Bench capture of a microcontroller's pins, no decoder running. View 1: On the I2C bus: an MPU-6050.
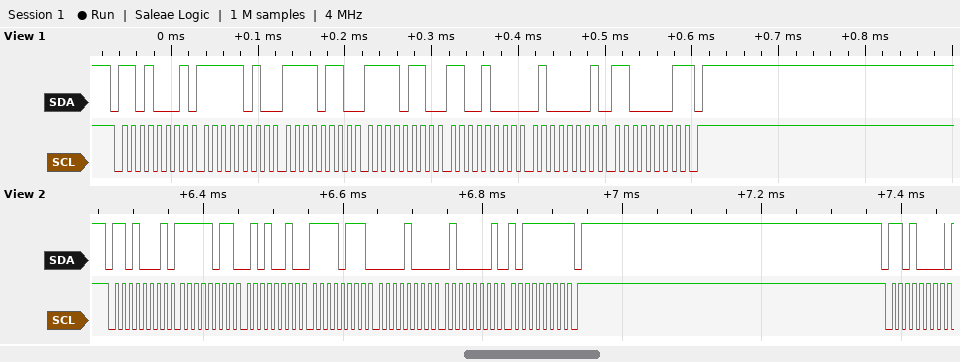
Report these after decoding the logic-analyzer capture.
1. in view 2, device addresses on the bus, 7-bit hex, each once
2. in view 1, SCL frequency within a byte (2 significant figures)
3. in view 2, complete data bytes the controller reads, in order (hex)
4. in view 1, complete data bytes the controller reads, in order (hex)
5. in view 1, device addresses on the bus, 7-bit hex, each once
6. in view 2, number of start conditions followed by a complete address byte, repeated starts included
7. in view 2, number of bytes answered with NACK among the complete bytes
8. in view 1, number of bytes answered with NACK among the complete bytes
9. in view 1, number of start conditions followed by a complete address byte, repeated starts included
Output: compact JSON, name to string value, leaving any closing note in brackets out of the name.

{"in view 2, device addresses on the bus, 7-bit hex, each once": "0x68", "in view 1, SCL frequency within a byte": "100 kHz", "in view 2, complete data bytes the controller reads, in order": "FB 52 F7 08 41 BF", "in view 1, complete data bytes the controller reads, in order": "FA F6 F6 C8 41 C1", "in view 1, device addresses on the bus, 7-bit hex, each once": "0x68", "in view 2, number of start conditions followed by a complete address byte, repeated starts included": "2", "in view 2, number of bytes answered with NACK among the complete bytes": "1", "in view 1, number of bytes answered with NACK among the complete bytes": "1", "in view 1, number of start conditions followed by a complete address byte, repeated starts included": "1"}
